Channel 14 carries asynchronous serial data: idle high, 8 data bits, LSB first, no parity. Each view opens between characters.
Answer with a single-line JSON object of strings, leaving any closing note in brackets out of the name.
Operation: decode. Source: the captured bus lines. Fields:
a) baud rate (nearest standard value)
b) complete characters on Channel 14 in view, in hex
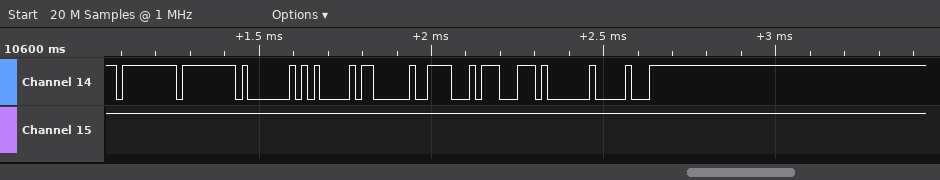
{"baud rate": "57600 baud", "complete characters on Channel 14 in view, in hex": "FF, FF, 01, 05, 03, 1E, C7, 01, 10"}
